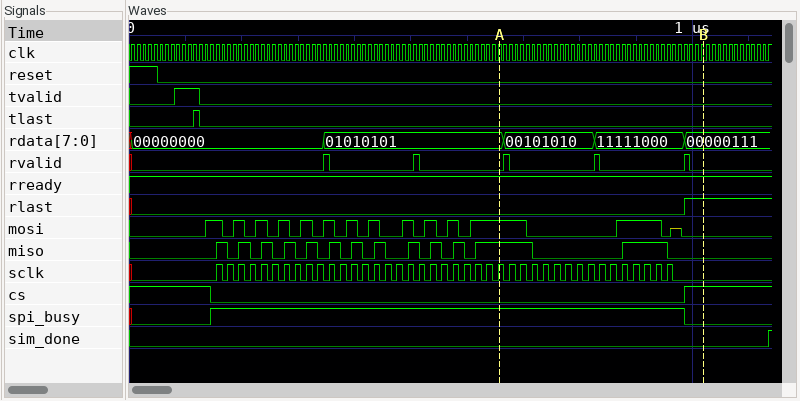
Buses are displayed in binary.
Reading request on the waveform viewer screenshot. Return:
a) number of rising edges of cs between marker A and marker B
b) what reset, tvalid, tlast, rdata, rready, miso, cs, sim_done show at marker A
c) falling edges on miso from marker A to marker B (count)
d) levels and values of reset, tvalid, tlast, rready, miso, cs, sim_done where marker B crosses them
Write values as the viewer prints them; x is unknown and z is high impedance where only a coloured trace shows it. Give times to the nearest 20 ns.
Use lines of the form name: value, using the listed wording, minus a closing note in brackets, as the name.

number of rising edges of cs between marker A and marker B: 1
what reset, tvalid, tlast, rdata, rready, miso, cs, sim_done show at marker A: reset=0, tvalid=0, tlast=0, rdata=01010101, rready=1, miso=1, cs=0, sim_done=0
falling edges on miso from marker A to marker B: 2
levels and values of reset, tvalid, tlast, rready, miso, cs, sim_done where marker B crosses them: reset=0, tvalid=0, tlast=0, rready=1, miso=0, cs=1, sim_done=0
